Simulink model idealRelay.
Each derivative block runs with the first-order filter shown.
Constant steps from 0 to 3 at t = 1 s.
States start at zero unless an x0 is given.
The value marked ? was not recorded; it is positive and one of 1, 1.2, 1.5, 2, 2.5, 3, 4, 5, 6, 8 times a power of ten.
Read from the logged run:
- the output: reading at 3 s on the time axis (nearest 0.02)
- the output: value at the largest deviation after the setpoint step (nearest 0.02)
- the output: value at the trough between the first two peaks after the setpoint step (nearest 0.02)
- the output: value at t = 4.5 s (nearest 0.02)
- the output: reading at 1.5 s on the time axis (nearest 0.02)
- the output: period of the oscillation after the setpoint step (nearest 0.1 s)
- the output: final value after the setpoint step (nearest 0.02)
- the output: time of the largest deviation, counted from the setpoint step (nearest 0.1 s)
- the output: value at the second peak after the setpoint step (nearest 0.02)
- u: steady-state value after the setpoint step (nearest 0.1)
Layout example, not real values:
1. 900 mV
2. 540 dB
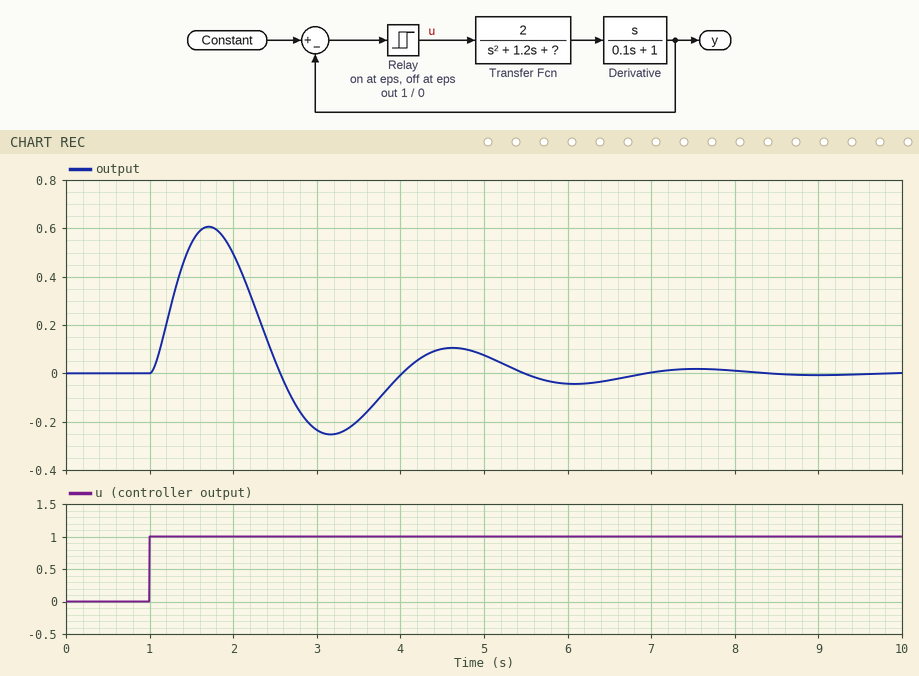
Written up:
1. -0.24
2. 0.60
3. -0.26
4. 0.10
5. 0.54
6. 2.9 s
7. 0.00
8. 0.7 s
9. 0.10
10. 1.0
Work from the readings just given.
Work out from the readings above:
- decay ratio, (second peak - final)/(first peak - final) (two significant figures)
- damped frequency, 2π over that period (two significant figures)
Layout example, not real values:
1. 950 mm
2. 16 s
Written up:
1. 0.17
2. 2.2 rad/s
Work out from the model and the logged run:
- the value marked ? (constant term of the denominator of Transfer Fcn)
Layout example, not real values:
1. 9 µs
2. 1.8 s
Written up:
1. 5
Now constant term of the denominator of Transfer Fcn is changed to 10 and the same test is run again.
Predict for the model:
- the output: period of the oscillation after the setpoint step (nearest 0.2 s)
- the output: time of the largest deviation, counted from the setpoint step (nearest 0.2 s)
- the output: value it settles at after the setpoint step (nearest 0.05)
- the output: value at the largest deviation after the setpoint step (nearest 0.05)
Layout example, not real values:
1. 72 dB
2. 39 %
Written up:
1. 2.0 s
2. 0.6 s
3. 0.00
4. 0.45
